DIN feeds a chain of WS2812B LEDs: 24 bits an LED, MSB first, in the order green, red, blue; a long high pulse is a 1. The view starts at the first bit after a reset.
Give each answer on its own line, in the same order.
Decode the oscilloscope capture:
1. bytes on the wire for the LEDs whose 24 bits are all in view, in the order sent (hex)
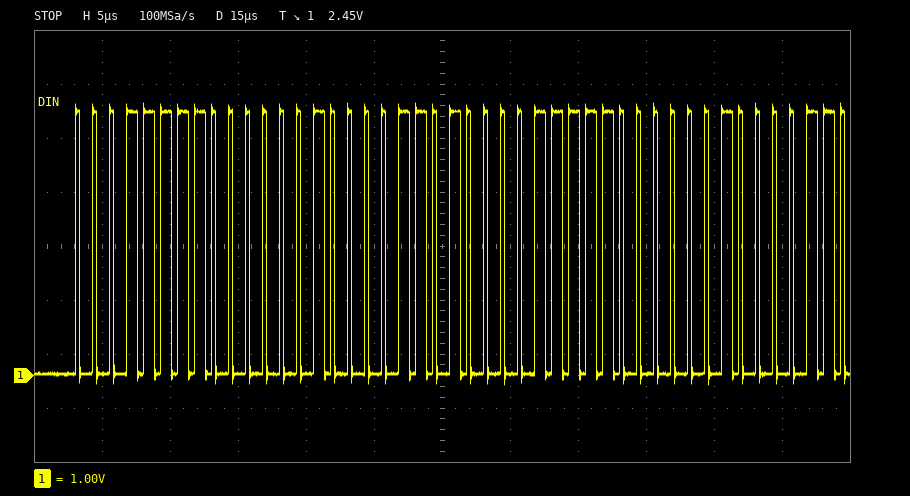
1F 02 1A
